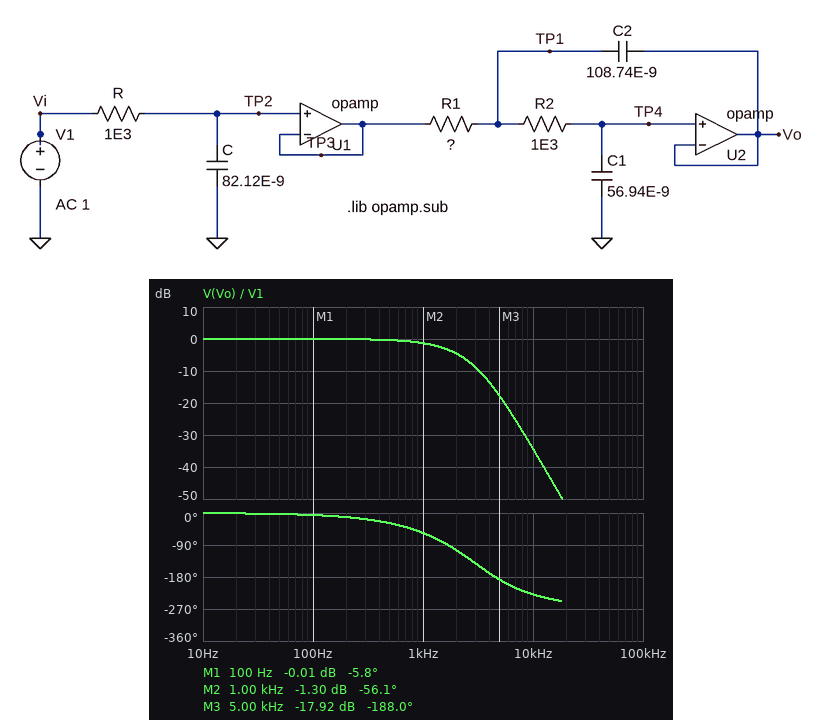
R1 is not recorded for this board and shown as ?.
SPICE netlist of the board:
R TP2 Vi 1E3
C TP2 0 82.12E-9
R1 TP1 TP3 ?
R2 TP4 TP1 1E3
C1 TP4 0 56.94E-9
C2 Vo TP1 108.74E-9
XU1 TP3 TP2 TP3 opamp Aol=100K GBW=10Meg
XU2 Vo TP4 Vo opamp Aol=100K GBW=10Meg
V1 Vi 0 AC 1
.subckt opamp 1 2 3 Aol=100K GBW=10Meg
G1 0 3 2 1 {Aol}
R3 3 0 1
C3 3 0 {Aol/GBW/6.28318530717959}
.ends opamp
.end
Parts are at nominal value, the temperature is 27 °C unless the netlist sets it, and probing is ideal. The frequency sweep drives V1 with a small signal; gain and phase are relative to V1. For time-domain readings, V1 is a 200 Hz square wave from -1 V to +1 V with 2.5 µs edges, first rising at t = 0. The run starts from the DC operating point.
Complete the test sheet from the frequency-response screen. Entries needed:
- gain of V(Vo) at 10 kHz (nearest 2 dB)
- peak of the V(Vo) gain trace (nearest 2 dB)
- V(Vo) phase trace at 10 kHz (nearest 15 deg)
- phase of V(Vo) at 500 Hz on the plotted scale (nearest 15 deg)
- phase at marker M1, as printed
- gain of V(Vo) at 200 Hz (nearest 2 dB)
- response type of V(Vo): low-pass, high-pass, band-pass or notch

-34 dB
0 dB
-225 deg
-30 deg
-5.8 deg
0 dB
low-pass
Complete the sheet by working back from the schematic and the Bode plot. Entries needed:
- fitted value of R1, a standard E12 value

390 Ω
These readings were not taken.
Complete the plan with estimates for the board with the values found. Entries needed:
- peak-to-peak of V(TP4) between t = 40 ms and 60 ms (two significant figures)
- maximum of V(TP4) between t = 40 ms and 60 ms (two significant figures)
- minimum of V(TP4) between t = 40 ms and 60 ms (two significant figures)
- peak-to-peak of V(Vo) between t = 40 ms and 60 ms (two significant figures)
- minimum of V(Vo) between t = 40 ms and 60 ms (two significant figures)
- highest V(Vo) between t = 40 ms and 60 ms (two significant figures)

2.0 V
1.0 V
-1.0 V
2.0 V
-1.0 V
1.0 V
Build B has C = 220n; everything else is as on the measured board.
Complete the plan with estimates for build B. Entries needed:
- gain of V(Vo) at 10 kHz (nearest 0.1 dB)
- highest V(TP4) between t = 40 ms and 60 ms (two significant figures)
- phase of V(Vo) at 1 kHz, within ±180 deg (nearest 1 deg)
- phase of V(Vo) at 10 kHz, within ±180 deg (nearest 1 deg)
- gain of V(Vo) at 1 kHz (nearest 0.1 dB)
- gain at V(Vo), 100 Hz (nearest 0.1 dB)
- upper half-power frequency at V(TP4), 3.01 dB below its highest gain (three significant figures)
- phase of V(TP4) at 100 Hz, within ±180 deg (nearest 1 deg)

-42.7 dB
1.0 V
-83 deg
124 deg
-4.9 dB
-0.1 dB
702 Hz
-11 deg
